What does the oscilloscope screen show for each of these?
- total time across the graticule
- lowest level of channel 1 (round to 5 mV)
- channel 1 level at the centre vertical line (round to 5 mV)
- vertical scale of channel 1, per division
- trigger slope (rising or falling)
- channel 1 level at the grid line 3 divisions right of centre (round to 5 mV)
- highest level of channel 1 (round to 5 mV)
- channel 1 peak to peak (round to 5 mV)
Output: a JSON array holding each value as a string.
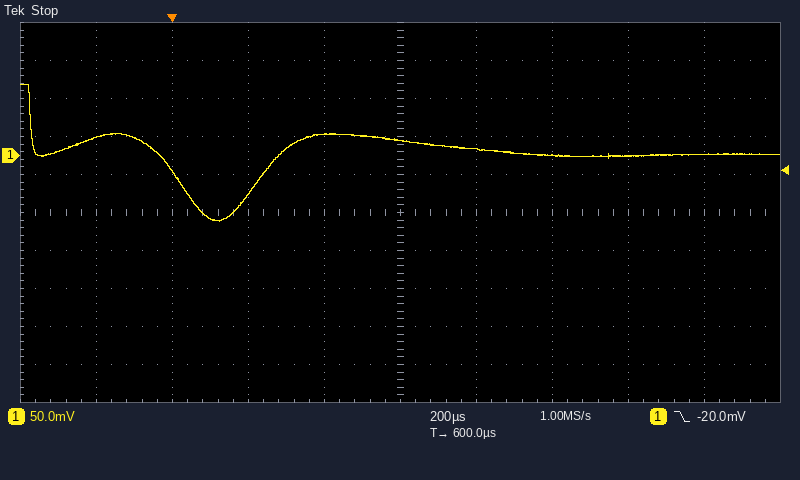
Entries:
["2 ms", "-85 mV", "20 mV", "50 mV", "falling", "0 mV", "95 mV", "180 mV"]
